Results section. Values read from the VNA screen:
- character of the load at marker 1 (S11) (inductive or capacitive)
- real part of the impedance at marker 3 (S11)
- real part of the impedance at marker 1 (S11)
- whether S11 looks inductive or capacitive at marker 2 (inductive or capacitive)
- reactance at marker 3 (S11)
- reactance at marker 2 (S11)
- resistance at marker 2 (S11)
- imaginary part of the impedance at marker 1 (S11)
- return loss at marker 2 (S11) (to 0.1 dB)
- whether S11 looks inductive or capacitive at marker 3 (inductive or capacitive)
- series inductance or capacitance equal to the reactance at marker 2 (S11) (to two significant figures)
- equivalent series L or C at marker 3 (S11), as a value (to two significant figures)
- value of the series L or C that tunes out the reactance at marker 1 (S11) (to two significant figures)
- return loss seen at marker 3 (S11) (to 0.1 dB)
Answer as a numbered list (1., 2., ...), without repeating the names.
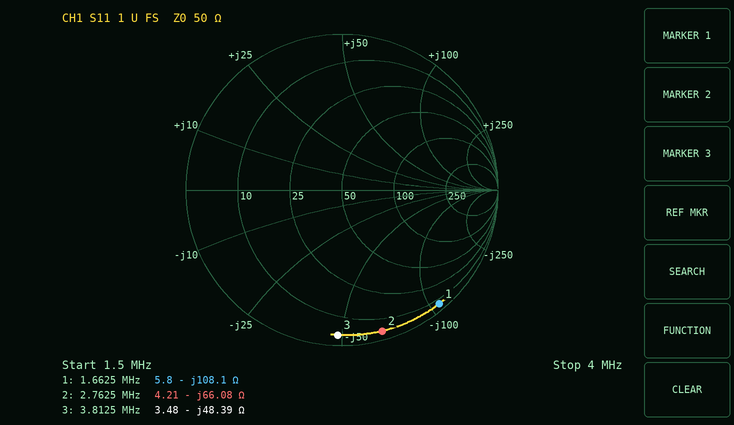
1. capacitive
2. 3.48 Ω
3. 5.8 Ω
4. capacitive
5. -48.39 Ω
6. -66.08 Ω
7. 4.21 Ω
8. -108.1 Ω
9. 0.5 dB
10. capacitive
11. 870 pF
12. 860 pF
13. 10 µH
14. 0.6 dB
